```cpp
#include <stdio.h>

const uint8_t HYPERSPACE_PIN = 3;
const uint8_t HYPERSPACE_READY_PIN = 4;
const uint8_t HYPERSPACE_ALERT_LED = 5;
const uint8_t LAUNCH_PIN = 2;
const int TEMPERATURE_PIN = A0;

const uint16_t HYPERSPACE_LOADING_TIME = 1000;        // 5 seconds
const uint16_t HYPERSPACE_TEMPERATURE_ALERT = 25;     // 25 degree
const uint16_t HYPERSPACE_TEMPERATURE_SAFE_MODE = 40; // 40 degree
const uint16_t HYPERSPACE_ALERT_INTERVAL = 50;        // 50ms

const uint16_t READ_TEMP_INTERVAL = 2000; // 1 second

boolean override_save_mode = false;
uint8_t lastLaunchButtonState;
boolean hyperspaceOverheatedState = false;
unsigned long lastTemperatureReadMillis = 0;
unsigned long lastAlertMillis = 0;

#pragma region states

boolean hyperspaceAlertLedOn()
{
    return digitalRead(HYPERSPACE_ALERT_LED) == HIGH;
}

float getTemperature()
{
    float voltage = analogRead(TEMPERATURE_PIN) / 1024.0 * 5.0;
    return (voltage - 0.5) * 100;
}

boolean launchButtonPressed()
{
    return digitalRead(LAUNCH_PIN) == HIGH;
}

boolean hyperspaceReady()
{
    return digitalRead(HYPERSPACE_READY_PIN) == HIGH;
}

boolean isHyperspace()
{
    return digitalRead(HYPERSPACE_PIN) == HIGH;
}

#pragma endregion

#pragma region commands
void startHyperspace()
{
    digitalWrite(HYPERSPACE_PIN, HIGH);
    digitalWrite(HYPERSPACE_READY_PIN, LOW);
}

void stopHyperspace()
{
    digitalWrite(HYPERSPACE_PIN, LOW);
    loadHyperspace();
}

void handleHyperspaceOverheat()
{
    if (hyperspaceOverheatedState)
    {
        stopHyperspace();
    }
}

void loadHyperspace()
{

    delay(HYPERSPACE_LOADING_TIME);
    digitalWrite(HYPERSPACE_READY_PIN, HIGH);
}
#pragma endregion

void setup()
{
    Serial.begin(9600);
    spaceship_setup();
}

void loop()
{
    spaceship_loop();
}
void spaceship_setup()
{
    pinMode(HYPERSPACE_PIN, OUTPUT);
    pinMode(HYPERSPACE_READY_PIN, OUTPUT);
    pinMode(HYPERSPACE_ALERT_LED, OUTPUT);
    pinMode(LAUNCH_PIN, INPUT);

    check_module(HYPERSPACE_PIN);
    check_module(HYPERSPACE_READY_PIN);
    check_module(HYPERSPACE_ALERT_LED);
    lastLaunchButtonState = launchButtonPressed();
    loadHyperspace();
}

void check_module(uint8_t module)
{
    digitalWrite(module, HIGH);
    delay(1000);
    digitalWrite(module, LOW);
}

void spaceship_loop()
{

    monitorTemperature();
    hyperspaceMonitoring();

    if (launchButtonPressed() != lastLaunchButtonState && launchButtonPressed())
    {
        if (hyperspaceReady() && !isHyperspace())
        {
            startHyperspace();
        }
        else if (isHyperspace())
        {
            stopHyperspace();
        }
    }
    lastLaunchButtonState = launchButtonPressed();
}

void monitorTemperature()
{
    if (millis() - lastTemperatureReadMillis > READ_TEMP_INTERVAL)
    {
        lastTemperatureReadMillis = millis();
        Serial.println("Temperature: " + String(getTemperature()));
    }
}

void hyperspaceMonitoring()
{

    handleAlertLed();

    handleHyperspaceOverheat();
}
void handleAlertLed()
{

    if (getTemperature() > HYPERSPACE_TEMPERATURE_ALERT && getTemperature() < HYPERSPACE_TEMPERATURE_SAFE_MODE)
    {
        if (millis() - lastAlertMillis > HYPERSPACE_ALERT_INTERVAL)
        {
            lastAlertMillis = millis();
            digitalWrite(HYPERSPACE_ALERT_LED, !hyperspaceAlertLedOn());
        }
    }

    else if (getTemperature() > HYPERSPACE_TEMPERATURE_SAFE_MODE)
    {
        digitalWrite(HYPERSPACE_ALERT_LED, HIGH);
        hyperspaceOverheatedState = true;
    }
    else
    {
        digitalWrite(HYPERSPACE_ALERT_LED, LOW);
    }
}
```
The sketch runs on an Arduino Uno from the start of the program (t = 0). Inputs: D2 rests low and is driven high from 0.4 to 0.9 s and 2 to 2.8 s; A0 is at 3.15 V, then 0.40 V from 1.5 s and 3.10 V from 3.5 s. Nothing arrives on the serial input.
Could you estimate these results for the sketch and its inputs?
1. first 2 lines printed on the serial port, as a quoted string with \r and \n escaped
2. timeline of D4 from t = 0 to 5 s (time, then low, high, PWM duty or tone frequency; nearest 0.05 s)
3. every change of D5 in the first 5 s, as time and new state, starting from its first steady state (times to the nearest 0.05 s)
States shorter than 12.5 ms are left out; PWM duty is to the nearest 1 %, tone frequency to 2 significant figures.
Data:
"Temperature: 259.57\r\nTemperature: 259.57\r\n"
0 s low; 1 s high; 2 s low; 4 s high
0 s low; 2 s high; 3 s low; 4 s high
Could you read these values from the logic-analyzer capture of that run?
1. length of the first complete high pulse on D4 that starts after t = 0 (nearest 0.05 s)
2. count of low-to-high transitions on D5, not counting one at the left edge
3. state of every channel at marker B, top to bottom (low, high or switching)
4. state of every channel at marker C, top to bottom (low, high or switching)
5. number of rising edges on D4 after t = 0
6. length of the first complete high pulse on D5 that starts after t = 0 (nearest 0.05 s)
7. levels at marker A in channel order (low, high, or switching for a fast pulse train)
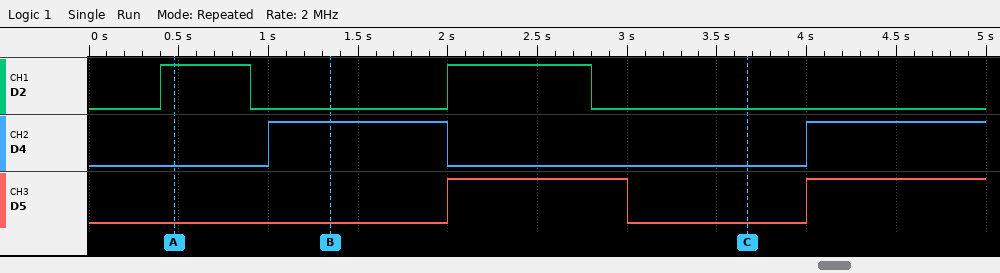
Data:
1.00 s
2
D2 low, D4 high, D5 low
D2 low, D4 low, D5 low
2
1.00 s
D2 high, D4 low, D5 low
